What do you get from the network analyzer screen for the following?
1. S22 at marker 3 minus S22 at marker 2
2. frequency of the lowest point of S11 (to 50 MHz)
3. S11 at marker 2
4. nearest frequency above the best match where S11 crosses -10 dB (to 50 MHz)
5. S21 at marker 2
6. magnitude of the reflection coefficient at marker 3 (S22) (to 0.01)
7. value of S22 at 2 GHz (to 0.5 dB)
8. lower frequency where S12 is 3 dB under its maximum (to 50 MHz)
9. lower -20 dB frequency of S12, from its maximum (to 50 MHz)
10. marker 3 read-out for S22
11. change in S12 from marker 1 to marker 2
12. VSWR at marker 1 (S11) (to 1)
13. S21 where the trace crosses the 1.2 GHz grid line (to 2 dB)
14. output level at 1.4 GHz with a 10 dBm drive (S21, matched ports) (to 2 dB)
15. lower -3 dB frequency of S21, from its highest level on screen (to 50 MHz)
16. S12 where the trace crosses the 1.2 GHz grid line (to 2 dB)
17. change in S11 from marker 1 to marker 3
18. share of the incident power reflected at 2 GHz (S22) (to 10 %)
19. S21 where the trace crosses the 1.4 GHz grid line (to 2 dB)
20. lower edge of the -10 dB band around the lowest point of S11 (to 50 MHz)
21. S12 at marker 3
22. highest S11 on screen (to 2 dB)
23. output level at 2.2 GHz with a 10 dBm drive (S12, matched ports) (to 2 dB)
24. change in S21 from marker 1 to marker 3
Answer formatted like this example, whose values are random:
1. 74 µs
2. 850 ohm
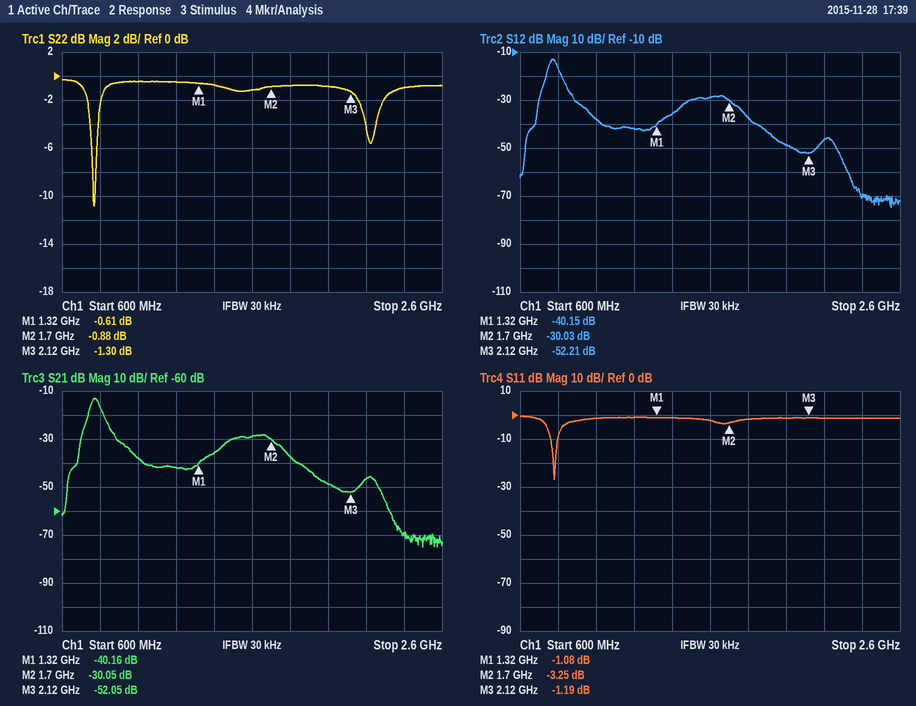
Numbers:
1. -0.42 dB
2. 800 MHz
3. -3.25 dB
4. 800 MHz
5. -30.05 dB
6. 0.86
7. -1.0 dB
8. 750 MHz
9. 700 MHz
10. -1.30 dB
11. 10.12 dB
12. 16
13. -42 dB
14. -26 dBm
15. 750 MHz
16. -42 dB
17. -0.11 dB
18. 80 %
19. -36 dB
20. 750 MHz
21. -52.21 dB
22. 0 dB
23. -36 dBm
24. -11.89 dB
